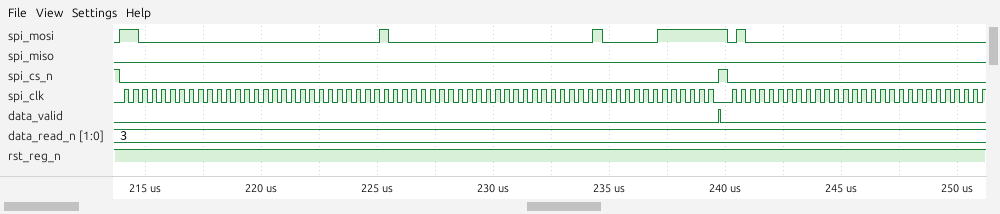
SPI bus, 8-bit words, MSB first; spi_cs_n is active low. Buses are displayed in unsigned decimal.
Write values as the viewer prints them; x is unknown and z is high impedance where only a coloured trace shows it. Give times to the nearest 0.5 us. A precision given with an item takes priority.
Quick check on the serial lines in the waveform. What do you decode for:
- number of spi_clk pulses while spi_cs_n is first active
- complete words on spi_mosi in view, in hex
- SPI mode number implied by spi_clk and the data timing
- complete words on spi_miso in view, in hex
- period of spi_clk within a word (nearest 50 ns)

64
C0, 00, 00, 08, 00, 00, 10, 3F, 40, 00, 00
0
00, 00, 00, 00, 00, 00, 00, 00, 00, 00, 00
400 ns
